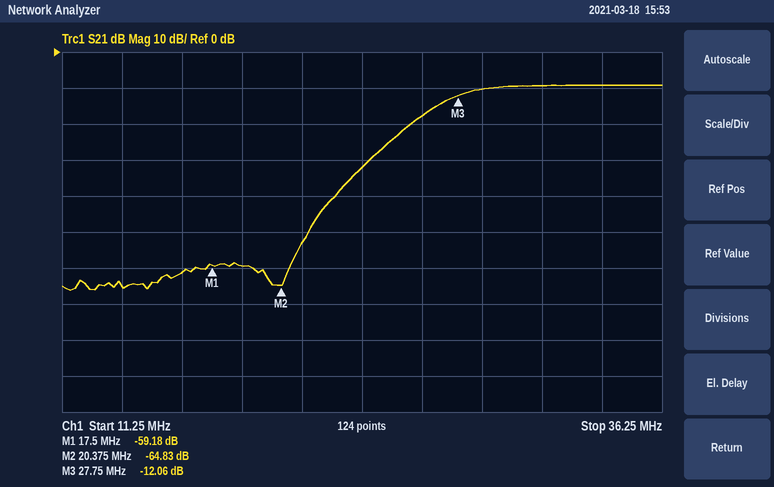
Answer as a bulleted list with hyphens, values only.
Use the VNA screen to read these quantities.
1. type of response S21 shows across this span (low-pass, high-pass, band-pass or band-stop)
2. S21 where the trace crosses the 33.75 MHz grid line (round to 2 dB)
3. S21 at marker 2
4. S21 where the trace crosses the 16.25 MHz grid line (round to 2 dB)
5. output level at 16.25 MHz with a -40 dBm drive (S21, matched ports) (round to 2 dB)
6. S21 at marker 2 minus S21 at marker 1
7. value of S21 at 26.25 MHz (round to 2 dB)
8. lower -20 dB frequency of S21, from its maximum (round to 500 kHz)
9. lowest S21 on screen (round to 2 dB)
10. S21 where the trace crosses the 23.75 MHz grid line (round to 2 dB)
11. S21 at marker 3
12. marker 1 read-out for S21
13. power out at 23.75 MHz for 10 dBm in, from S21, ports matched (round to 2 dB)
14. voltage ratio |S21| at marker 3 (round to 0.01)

- high-pass
- -10 dB
- -64.83 dB
- -62 dB
- -102 dBm
- -5.65 dB
- -18 dB
- 24.0 MHz
- -66 dB
- -32 dB
- -12.06 dB
- -59.18 dB
- -22 dBm
- 0.25
